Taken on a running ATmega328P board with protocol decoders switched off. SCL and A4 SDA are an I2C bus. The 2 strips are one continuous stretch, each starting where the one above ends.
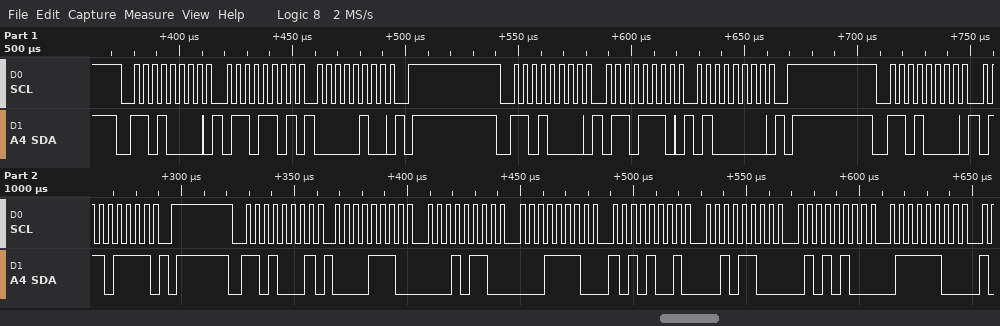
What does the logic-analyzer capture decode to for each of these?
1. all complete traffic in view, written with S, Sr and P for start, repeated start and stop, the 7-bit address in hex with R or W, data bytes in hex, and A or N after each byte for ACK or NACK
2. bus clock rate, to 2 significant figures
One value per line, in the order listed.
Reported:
S 68W A 6D A 04 A P S 68W A 6E A 40 A P S 68W A 6F A P S 68R A 0E A 16 A 1E A A9 A 2C A 54 A 7C A
250 kHz
